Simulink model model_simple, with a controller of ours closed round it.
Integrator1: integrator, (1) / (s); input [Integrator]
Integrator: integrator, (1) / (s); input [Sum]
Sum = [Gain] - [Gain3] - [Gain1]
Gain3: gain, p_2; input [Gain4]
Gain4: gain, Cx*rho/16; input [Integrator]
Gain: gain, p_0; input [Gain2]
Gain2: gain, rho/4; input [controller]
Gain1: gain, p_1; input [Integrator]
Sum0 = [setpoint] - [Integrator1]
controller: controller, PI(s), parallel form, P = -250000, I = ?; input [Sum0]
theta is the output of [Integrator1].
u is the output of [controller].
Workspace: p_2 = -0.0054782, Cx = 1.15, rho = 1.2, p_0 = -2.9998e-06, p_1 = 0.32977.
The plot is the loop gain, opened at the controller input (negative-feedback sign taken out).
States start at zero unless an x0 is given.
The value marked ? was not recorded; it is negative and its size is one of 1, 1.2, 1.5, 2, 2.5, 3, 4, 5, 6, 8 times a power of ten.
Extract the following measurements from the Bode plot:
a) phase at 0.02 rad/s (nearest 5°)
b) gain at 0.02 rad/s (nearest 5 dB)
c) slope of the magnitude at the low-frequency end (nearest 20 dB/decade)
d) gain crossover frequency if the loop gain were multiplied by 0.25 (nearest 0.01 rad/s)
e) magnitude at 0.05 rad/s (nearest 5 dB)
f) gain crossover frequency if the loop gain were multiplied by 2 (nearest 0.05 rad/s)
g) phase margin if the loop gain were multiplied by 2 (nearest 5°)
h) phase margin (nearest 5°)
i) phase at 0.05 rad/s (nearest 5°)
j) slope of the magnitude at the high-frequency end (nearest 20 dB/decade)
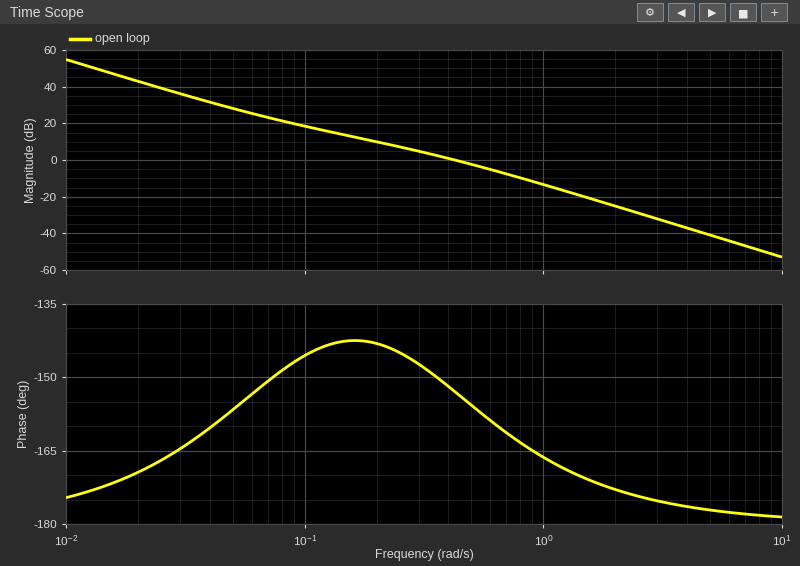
-170°
45 dB
-40 dB/decade
0.17 rad/s
30 dB
0.65 rad/s
20°
25°
-155°
-40 dB/decade
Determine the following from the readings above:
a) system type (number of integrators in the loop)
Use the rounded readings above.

2
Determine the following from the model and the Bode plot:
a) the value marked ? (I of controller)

-20000
